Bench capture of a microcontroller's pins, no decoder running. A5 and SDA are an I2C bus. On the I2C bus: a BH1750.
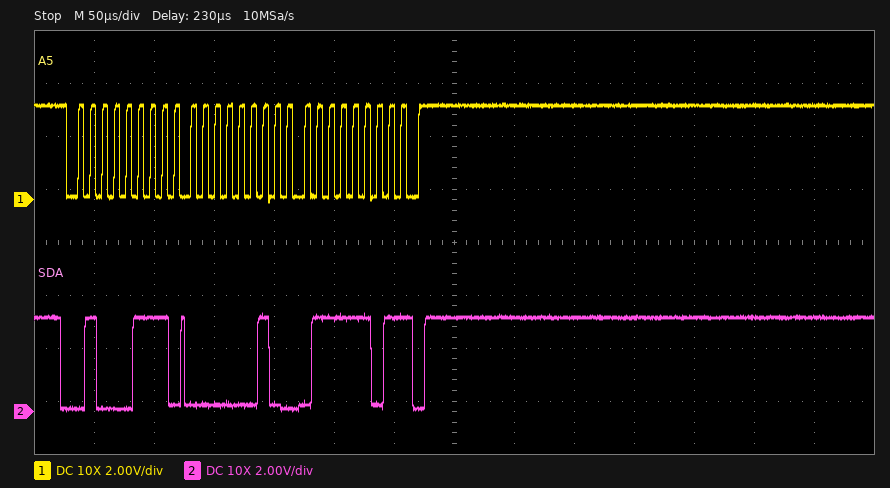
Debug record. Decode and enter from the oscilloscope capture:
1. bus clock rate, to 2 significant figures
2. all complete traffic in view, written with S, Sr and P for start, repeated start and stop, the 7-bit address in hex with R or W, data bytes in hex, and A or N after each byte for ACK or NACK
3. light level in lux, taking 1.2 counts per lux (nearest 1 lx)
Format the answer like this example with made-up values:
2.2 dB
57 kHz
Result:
100 kHz
S 23R A 02 A 7D N P
531 lx
